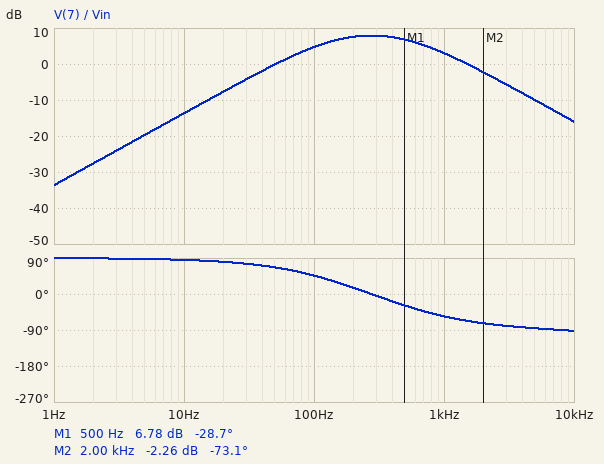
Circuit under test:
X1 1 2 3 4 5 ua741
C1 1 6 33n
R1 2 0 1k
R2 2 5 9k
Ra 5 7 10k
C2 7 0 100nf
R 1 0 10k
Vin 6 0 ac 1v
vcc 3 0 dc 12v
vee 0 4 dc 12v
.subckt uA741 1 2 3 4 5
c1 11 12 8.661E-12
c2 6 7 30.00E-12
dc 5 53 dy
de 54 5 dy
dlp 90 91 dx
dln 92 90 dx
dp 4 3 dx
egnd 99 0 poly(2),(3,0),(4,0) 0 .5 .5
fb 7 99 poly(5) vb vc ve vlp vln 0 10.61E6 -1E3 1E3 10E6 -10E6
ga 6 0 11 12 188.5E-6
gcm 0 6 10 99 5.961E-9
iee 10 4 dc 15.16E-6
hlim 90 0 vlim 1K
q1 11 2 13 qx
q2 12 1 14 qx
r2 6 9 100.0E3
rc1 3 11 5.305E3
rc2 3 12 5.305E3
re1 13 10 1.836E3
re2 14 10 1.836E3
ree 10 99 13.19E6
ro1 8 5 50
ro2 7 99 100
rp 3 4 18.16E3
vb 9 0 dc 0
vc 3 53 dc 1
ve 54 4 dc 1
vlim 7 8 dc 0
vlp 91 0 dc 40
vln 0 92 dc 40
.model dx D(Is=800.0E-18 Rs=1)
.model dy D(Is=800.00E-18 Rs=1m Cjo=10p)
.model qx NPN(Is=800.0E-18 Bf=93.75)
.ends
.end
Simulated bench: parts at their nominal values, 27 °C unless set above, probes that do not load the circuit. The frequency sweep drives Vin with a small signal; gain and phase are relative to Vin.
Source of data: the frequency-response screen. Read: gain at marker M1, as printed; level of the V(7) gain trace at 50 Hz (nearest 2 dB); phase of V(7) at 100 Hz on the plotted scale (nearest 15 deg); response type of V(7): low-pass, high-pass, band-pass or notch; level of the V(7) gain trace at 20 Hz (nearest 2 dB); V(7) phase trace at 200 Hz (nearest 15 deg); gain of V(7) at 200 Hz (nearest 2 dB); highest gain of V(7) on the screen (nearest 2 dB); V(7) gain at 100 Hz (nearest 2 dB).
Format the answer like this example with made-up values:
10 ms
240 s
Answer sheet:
6.78 dB
0 dB
45 deg
band-pass
-8 dB
15 deg
8 dB
8 dB
4 dB
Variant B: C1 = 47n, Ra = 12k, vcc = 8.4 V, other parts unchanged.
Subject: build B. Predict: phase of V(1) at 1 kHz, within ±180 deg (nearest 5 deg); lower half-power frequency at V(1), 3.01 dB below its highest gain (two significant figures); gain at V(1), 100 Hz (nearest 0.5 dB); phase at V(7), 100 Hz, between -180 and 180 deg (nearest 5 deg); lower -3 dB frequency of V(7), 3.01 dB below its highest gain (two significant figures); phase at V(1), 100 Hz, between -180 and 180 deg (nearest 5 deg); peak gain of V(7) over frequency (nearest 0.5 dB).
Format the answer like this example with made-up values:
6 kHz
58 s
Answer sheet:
20 deg
340 Hz
-11.0 dB
35 deg
81 Hz
75 deg
9.0 dB
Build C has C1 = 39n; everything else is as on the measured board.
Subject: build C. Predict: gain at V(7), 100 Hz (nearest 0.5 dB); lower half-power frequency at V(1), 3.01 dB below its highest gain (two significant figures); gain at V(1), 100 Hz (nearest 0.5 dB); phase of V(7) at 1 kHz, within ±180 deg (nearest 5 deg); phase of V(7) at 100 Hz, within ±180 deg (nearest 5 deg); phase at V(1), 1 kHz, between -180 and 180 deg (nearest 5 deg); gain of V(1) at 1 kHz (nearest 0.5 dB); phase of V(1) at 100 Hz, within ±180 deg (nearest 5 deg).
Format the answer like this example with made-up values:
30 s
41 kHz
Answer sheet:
6.0 dB
410 Hz
-12.5 dB
-60 deg
45 deg
20 deg
-0.5 dB
75 deg
